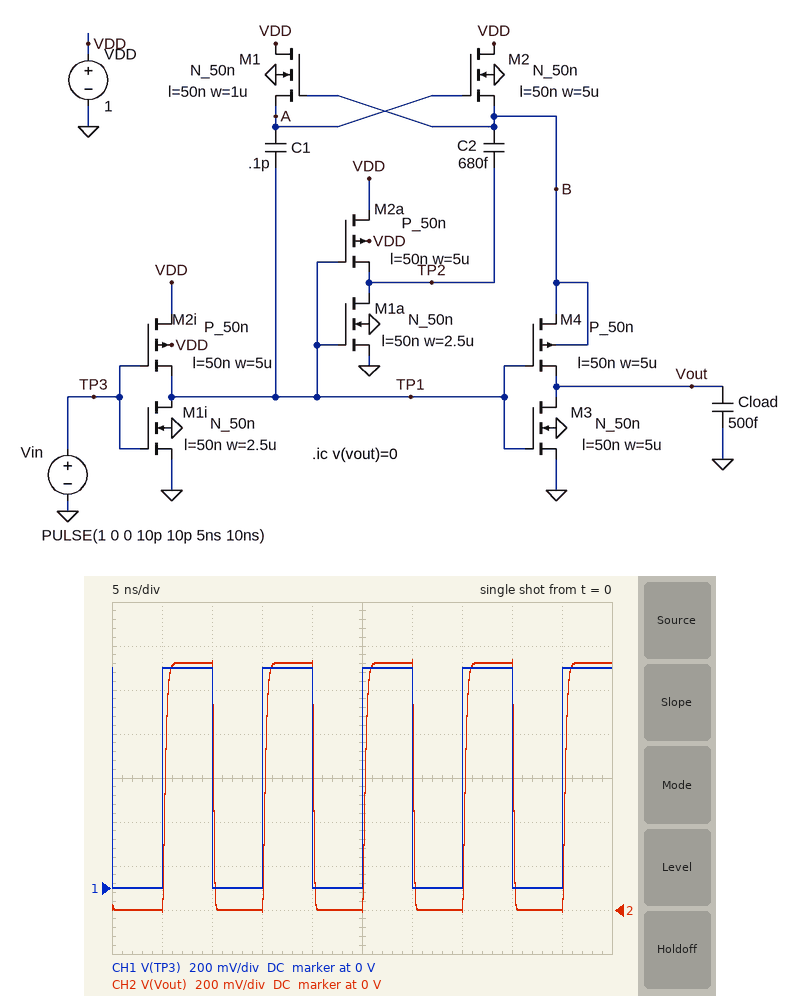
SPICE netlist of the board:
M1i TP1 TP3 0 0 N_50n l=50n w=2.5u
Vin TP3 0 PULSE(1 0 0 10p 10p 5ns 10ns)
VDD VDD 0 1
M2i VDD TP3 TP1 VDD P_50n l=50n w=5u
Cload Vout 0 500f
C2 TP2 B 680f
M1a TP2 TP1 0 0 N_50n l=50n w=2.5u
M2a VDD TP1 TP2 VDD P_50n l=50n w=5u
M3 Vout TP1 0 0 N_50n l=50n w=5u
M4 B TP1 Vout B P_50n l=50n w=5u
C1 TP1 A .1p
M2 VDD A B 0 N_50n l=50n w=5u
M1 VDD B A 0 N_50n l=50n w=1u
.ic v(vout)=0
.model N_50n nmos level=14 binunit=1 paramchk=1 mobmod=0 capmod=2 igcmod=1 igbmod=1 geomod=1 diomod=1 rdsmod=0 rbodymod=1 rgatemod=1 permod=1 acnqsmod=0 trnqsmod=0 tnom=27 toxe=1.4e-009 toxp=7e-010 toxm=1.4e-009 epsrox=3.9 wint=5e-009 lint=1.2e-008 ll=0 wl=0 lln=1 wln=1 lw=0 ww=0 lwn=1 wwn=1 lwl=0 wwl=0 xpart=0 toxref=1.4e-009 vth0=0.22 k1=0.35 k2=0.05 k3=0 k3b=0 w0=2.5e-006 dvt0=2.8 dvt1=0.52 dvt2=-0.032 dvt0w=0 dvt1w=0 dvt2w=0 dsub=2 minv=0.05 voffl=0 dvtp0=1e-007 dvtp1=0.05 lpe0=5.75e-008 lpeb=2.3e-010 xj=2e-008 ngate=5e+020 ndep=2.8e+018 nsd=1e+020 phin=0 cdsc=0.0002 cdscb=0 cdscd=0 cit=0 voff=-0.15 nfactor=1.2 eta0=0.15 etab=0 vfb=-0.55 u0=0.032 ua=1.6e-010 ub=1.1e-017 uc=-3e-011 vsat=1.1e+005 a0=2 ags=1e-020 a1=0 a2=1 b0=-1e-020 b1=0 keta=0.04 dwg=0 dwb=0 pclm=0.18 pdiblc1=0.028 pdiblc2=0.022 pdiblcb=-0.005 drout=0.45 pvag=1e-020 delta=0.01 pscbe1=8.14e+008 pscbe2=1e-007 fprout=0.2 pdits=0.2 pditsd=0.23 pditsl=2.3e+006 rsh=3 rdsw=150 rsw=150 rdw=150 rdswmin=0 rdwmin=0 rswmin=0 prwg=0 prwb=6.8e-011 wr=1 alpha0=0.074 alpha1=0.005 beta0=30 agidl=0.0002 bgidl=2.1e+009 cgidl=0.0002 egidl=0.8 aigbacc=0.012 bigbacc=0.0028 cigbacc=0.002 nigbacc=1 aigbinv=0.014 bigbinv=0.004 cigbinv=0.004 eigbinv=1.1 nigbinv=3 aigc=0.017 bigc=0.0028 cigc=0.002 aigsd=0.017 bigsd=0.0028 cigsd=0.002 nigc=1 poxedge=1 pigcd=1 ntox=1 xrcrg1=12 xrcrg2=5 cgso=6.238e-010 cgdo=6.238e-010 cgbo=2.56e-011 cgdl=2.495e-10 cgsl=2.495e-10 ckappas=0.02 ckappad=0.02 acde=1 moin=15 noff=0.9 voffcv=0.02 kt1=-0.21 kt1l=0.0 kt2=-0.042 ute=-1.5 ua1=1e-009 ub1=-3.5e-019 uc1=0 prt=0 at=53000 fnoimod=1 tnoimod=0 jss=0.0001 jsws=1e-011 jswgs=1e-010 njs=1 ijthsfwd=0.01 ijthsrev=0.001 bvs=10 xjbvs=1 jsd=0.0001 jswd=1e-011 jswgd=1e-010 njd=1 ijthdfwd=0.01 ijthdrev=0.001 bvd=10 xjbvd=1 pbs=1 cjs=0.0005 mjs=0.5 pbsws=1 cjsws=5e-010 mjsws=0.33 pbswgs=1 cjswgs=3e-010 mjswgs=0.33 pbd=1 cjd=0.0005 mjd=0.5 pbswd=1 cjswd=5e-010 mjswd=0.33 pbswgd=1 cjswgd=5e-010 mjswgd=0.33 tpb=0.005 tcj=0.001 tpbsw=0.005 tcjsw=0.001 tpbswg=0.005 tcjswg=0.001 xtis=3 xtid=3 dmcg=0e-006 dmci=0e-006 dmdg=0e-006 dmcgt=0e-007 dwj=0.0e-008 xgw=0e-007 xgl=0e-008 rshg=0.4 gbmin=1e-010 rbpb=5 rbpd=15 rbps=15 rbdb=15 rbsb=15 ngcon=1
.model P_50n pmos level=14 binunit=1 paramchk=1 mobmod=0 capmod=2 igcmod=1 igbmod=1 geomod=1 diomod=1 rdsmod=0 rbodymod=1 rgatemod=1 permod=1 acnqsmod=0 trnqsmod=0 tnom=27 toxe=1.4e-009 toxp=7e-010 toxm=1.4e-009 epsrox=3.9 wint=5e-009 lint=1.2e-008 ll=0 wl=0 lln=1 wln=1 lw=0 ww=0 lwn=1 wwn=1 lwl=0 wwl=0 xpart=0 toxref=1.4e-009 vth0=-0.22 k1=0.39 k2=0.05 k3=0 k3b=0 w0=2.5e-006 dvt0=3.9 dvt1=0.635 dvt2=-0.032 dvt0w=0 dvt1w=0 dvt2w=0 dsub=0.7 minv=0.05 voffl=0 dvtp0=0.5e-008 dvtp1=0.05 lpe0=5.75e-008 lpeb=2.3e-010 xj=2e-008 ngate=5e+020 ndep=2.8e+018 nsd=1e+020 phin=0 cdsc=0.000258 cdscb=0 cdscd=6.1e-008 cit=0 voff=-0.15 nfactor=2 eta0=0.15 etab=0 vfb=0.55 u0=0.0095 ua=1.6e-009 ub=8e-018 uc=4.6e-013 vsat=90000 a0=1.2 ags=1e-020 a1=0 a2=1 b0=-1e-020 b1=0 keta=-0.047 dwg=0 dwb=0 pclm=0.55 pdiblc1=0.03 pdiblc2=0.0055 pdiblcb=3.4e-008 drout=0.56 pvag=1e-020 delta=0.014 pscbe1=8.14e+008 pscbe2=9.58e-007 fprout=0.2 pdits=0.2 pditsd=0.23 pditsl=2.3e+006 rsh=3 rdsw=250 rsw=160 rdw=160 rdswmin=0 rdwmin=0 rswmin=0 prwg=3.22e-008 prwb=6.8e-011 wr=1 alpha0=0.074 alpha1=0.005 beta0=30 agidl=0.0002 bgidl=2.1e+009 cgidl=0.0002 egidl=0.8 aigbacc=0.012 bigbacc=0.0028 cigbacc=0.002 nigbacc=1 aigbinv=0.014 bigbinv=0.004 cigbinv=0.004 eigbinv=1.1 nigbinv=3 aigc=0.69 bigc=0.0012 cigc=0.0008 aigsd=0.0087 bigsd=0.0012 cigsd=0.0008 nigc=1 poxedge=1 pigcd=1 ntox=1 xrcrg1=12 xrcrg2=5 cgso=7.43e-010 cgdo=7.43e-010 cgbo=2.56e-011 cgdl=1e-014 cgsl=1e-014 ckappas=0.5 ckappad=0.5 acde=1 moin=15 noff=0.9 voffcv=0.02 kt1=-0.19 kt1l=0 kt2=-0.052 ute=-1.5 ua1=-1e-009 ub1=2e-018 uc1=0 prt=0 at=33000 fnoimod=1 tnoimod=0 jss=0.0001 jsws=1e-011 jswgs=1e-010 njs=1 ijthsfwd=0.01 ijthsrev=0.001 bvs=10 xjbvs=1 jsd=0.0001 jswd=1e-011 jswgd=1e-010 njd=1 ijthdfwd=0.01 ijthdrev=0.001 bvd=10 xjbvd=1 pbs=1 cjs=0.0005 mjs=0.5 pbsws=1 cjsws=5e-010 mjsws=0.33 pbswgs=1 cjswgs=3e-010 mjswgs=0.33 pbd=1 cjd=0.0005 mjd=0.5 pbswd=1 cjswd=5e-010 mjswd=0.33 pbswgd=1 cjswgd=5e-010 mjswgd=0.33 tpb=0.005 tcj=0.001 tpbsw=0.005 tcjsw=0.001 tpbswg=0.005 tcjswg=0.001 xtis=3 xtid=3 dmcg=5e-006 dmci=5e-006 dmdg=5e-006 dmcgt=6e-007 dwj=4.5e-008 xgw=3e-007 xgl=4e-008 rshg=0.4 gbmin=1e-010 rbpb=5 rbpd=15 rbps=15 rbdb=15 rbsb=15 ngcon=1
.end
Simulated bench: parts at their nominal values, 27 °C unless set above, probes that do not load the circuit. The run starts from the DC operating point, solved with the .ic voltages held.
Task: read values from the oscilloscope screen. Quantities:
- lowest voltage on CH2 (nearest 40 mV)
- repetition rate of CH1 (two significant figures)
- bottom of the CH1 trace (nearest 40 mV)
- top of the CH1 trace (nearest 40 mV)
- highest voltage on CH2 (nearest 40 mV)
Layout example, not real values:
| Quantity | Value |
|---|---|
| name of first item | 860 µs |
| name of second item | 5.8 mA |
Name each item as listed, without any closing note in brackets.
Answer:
| Quantity | Value |
|---|---|
| lowest voltage on CH2 | 0 V |
| repetition rate of CH1 | 100 MHz |
| bottom of the CH1 trace | 0 V |
| top of the CH1 trace | 1.00 V |
| highest voltage on CH2 | 1.12 V |
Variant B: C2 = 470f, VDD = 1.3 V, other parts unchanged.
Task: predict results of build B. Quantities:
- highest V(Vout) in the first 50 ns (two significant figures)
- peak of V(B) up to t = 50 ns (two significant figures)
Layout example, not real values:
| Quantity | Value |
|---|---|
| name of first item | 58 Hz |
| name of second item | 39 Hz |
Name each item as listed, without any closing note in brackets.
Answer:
| Quantity | Value |
|---|---|
| highest V(Vout) in the first 50 ns | 1.2 V |
| peak of V(B) up to t = 50 ns | 1.3 V |
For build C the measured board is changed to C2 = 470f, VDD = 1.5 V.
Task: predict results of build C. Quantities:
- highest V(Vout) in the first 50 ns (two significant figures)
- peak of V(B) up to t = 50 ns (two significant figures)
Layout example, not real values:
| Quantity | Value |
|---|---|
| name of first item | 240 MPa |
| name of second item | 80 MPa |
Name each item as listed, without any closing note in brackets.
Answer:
| Quantity | Value |
|---|---|
| highest V(Vout) in the first 50 ns | 1.4 V |
| peak of V(B) up to t = 50 ns | 1.5 V |
